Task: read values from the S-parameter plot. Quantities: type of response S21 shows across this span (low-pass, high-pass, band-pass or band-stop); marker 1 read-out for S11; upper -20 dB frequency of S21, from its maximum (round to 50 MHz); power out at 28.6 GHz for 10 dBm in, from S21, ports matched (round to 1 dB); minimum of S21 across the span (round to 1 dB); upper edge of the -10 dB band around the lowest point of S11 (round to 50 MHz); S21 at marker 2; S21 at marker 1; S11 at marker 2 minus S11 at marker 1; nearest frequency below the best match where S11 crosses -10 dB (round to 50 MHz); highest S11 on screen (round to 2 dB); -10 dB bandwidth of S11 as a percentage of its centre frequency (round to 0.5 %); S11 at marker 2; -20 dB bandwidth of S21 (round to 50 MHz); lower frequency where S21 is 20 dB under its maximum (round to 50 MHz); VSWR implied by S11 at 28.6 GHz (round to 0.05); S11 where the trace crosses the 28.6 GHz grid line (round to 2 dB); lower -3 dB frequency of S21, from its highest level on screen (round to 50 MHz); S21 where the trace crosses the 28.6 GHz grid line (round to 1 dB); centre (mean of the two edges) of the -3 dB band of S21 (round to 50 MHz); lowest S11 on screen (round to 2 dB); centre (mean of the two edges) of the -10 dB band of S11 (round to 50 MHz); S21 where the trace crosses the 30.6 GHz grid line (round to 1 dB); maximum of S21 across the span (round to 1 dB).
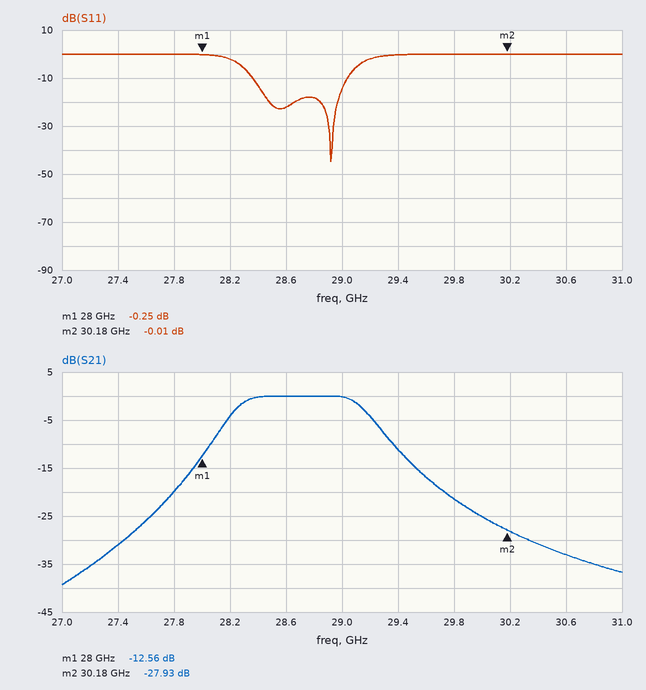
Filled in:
band-pass
-0.25 dB
29.75 GHz
10 dBm
-39 dB
29.05 GHz
-27.93 dB
-12.56 dB
0.24 dB
28.35 GHz
0 dB
2.5 %
-0.01 dB
1.95 GHz
27.80 GHz
1.15
-22 dB
28.25 GHz
0 dB
28.70 GHz
-44 dB
28.70 GHz
-33 dB
0 dB
